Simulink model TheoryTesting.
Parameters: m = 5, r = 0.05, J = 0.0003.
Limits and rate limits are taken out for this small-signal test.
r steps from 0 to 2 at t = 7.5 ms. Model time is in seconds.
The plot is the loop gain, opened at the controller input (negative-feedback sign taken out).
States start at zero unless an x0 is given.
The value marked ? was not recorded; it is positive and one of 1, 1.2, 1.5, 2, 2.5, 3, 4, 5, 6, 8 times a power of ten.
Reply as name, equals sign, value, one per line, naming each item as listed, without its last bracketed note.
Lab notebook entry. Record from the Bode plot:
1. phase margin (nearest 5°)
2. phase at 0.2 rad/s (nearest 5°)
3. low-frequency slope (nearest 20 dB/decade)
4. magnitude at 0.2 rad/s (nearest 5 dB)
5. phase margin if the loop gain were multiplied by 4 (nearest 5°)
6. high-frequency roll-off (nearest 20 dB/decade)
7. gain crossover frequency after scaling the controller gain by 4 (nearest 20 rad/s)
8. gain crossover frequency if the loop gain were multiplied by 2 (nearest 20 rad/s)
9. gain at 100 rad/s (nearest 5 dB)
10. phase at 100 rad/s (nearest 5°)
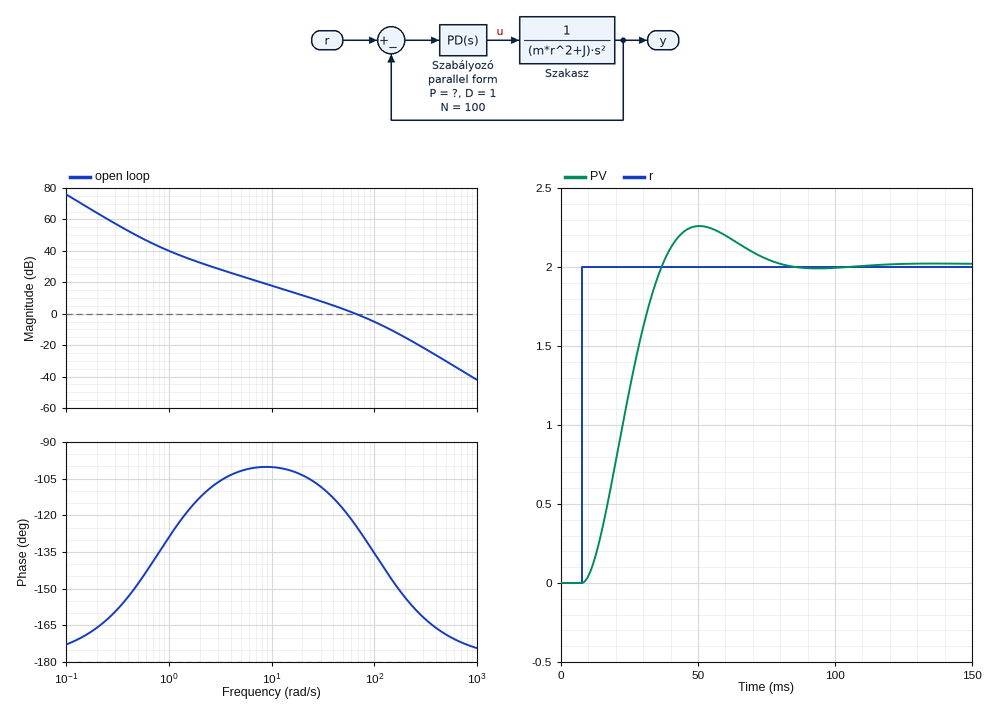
phase margin = 55°
phase at 0.2 rad/s = -165°
low-frequency slope = -40 dB/decade
magnitude at 0.2 rad/s = 65 dB
phase margin if the loop gain were multiplied by 4 = 30°
high-frequency roll-off = -40 dB/decade
gain crossover frequency after scaling the controller gain by 4 = 160 rad/s
gain crossover frequency if the loop gain were multiplied by 2 = 100 rad/s
gain at 100 rad/s = -5 dB
phase at 100 rad/s = -135°
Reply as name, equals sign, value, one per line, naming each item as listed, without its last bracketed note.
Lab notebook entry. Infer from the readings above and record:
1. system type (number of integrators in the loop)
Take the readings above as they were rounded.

system type = 2
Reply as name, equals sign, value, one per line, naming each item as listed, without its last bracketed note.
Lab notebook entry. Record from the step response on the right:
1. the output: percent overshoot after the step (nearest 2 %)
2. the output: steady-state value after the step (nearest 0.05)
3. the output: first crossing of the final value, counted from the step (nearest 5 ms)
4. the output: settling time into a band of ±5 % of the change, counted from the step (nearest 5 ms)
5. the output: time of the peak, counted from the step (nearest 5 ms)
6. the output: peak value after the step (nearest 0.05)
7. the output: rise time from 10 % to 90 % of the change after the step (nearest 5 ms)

the output: percent overshoot after the step = 12 %
the output: steady-state value after the step = 2.00
the output: first crossing of the final value, counted from the step = 30 ms
the output: settling time into a band of ±5 % of the change, counted from the step = 60 ms
the output: time of the peak, counted from the step = 45 ms
the output: peak value after the step = 2.25
the output: rise time from 10 % to 90 % of the change after the step = 20 ms
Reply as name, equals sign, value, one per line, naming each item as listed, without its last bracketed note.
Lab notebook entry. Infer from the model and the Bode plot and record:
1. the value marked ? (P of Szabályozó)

the value marked ? = 0.8
